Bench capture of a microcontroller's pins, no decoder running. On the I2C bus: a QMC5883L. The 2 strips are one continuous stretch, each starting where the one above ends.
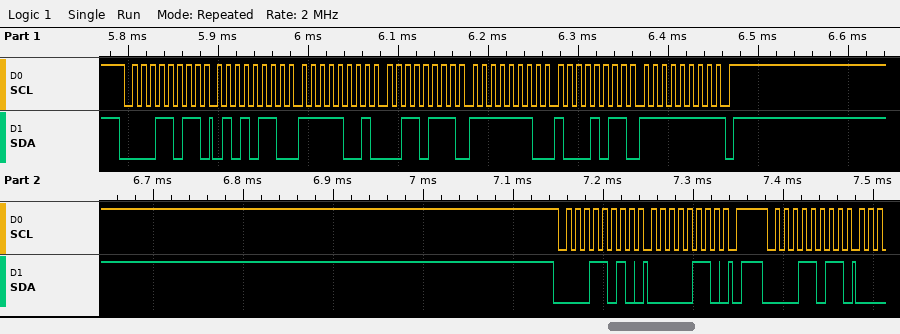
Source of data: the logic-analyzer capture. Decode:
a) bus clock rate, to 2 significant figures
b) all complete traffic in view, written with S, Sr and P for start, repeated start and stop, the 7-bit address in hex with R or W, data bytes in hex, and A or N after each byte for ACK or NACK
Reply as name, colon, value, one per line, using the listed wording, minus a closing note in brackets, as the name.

bus clock rate, to 2 significant figures: 100 kHz
all complete traffic in view, written with S, Sr and P for start, repeated start and stop, the 7-bit address in hex with R or W, data bytes in hex, and A or N after each byte for ACK or NACK: S 0DR A 56 A F9 A 37 A FE A 8B A FF N P S 0DW A 06 A P S 0DR A
